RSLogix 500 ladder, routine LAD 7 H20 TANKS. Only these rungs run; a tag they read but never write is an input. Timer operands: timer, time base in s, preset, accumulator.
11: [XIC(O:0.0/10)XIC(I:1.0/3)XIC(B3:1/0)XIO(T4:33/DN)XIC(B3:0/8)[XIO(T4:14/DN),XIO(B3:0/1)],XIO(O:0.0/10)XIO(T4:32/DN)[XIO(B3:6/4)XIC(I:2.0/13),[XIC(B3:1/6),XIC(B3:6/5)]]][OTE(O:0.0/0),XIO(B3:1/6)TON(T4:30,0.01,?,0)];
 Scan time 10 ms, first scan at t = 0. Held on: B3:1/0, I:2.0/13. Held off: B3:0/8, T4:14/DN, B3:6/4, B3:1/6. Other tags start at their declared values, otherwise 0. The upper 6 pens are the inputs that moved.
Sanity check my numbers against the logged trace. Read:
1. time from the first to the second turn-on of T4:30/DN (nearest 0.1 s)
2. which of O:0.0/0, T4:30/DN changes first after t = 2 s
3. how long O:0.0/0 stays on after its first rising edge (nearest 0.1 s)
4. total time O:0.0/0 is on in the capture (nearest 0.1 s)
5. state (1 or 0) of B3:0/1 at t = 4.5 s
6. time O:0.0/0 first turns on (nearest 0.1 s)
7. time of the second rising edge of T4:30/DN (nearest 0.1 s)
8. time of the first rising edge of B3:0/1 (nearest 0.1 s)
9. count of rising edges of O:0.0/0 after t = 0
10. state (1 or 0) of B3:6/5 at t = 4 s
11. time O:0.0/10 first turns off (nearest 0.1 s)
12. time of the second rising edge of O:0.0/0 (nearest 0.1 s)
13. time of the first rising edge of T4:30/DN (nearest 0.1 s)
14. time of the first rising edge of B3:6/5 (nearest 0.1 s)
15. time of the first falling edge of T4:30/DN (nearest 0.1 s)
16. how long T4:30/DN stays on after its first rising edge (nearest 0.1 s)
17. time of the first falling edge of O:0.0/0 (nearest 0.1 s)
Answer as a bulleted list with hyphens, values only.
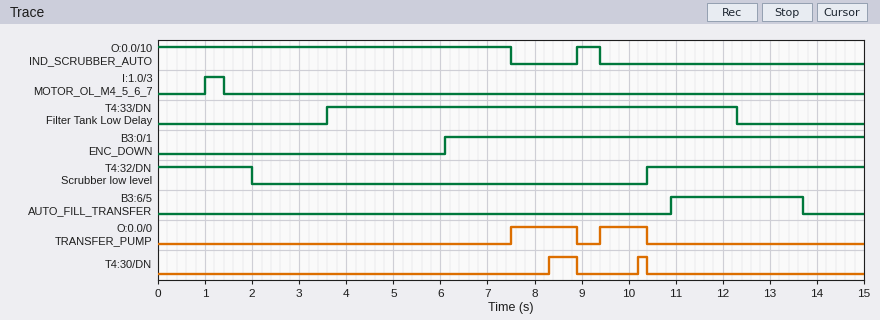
- 1.9 s
- O:0.0/0
- 1.4 s
- 2.4 s
- 0
- 7.5 s
- 10.2 s
- 6.1 s
- 2
- 0
- 7.5 s
- 9.4 s
- 8.3 s
- 10.9 s
- 8.9 s
- 0.6 s
- 8.9 s
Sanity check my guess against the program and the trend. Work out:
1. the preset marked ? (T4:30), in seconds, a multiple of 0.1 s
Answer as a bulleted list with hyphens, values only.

- 0.8 s
